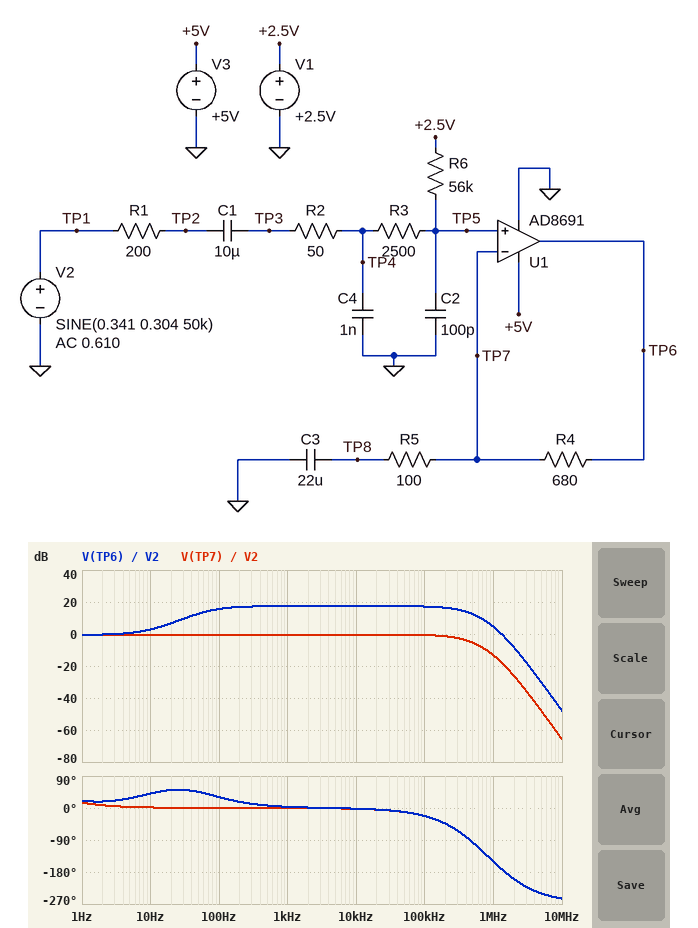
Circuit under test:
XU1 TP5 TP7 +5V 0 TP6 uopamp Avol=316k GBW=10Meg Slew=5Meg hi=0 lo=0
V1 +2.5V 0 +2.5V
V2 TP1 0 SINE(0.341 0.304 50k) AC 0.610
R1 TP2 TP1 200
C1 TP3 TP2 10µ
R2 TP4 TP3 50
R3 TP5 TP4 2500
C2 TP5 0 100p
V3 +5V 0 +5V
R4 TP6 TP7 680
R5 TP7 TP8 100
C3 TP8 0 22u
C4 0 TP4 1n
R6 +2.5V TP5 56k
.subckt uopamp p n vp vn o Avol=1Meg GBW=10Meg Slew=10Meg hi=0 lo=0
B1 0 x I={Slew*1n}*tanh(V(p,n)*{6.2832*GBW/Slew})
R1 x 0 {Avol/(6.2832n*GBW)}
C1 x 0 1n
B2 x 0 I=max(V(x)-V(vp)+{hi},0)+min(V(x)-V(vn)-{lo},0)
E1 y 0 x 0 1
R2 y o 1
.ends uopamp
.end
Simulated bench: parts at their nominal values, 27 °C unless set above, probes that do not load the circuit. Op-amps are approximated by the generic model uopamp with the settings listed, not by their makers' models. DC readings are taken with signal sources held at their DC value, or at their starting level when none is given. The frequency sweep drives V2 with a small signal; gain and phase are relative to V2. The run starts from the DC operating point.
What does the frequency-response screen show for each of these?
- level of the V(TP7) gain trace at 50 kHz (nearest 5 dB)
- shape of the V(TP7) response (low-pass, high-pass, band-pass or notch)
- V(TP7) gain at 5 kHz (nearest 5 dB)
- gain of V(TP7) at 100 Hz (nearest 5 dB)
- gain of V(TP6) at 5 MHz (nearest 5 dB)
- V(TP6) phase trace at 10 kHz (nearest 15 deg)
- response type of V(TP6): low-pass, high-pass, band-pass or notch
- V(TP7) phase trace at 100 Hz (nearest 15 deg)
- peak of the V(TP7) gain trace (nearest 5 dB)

0 dB
low-pass
0 dB
0 dB
-30 dB
0 deg
band-pass
0 deg
0 dB
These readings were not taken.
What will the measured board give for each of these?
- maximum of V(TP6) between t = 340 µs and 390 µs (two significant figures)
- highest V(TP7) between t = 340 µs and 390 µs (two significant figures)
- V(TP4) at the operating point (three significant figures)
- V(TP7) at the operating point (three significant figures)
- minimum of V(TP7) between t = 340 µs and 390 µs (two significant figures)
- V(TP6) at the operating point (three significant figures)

4.7 V
2.8 V
2.50 V
2.50 V
2.2 V
2.50 V
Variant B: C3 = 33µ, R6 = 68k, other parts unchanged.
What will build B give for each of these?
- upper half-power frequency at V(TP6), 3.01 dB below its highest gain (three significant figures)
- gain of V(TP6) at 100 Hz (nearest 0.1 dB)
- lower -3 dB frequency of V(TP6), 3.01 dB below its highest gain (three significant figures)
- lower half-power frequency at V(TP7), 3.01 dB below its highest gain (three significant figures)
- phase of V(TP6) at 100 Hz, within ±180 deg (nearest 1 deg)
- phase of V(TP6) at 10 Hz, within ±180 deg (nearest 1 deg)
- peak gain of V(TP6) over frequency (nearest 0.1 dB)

364 kHz
16.6 dB
47.4 Hz
225 mHz
22 deg
48 deg
17.5 dB
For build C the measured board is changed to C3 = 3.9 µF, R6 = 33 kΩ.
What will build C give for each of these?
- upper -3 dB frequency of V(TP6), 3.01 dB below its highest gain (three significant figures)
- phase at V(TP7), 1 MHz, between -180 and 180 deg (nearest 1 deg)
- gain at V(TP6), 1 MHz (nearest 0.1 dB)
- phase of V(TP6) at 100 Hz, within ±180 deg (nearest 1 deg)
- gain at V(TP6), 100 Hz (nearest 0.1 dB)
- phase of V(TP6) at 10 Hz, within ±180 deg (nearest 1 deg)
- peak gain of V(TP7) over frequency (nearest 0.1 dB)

372 kHz
-150 deg
4.4 dB
49 deg
5.7 dB
12 deg
-0.7 dB
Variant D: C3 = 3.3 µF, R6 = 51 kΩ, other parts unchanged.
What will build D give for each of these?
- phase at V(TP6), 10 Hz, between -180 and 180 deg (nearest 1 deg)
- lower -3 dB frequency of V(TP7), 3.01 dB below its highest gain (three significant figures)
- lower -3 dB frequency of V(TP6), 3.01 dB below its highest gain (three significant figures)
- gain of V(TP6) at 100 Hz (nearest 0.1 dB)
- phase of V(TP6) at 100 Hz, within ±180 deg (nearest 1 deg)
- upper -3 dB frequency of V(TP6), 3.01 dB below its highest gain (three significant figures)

10 deg
296 mHz
473 Hz
4.9 dB
47 deg
367 kHz
